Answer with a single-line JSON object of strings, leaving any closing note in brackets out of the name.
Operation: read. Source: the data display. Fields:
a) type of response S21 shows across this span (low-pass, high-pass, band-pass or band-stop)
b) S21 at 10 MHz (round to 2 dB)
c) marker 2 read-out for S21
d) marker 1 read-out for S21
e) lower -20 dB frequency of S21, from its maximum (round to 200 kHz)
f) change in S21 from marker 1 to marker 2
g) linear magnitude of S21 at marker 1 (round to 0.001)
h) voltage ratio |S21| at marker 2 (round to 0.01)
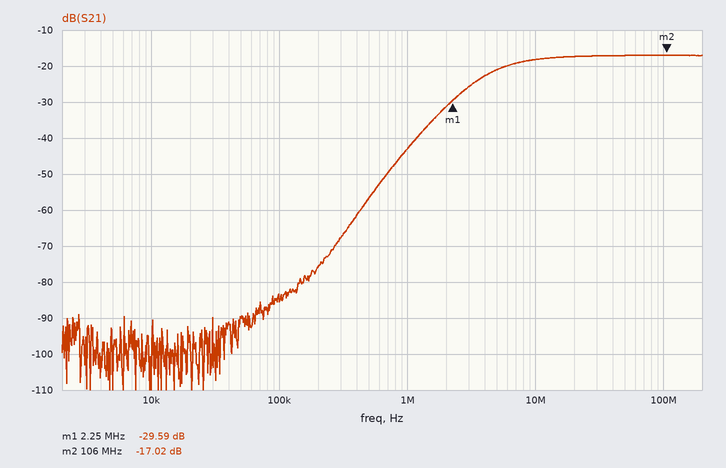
{"type of response S21 shows across this span": "high-pass", "S21 at 10 MHz": "-18 dB", "marker 2 read-out for S21": "-17.02 dB", "marker 1 read-out for S21": "-29.59 dB", "lower -20 dB frequency of S21, from its maximum": "1.4 MHz", "change in S21 from marker 1 to marker 2": "12.57 dB", "linear magnitude of S21 at marker 1": "0.033", "voltage ratio |S21| at marker 2": "0.14"}
